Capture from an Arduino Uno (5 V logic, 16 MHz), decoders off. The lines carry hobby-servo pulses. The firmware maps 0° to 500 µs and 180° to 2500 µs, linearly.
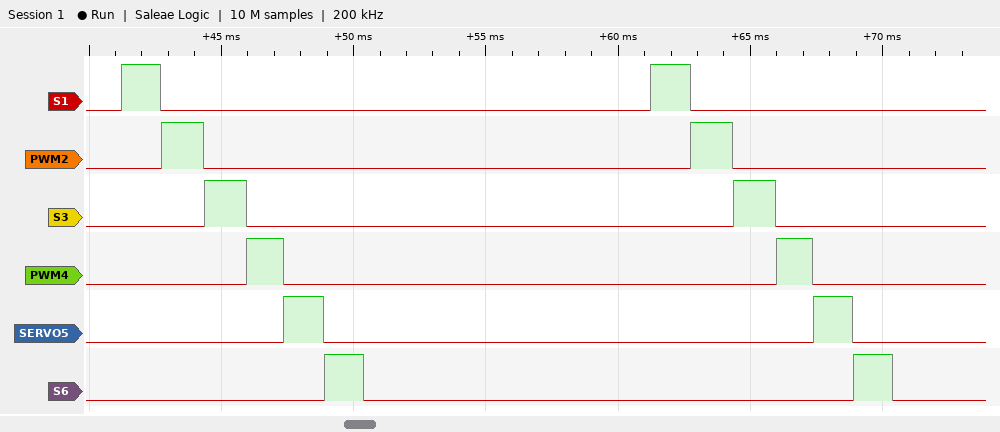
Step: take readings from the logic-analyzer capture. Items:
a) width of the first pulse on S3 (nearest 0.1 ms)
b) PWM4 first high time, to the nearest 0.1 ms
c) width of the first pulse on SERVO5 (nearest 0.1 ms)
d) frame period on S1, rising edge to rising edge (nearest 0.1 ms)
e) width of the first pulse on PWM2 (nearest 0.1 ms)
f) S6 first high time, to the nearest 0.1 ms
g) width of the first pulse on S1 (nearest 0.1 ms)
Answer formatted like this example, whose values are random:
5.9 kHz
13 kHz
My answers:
1.6 ms
1.4 ms
1.5 ms
20.0 ms
1.6 ms
1.5 ms
1.5 ms
